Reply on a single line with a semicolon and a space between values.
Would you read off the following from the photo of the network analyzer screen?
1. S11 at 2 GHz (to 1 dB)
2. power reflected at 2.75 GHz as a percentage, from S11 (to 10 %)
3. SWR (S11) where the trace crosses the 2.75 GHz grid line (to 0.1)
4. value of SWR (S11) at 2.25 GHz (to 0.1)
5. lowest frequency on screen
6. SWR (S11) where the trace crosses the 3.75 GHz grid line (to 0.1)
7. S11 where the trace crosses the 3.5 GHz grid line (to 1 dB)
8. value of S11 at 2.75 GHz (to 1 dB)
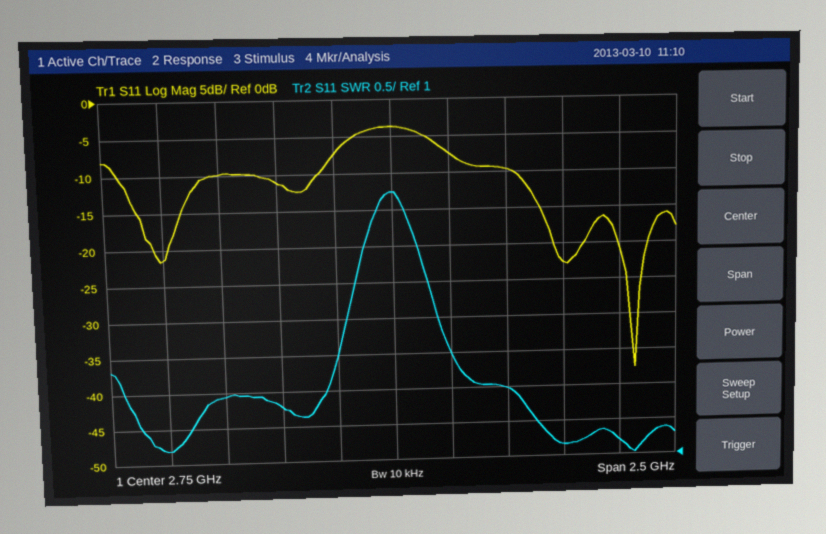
-10 dB; 40 %; 4.7; 1.8; 1.5 GHz; 1.2; -23 dB; -4 dB
